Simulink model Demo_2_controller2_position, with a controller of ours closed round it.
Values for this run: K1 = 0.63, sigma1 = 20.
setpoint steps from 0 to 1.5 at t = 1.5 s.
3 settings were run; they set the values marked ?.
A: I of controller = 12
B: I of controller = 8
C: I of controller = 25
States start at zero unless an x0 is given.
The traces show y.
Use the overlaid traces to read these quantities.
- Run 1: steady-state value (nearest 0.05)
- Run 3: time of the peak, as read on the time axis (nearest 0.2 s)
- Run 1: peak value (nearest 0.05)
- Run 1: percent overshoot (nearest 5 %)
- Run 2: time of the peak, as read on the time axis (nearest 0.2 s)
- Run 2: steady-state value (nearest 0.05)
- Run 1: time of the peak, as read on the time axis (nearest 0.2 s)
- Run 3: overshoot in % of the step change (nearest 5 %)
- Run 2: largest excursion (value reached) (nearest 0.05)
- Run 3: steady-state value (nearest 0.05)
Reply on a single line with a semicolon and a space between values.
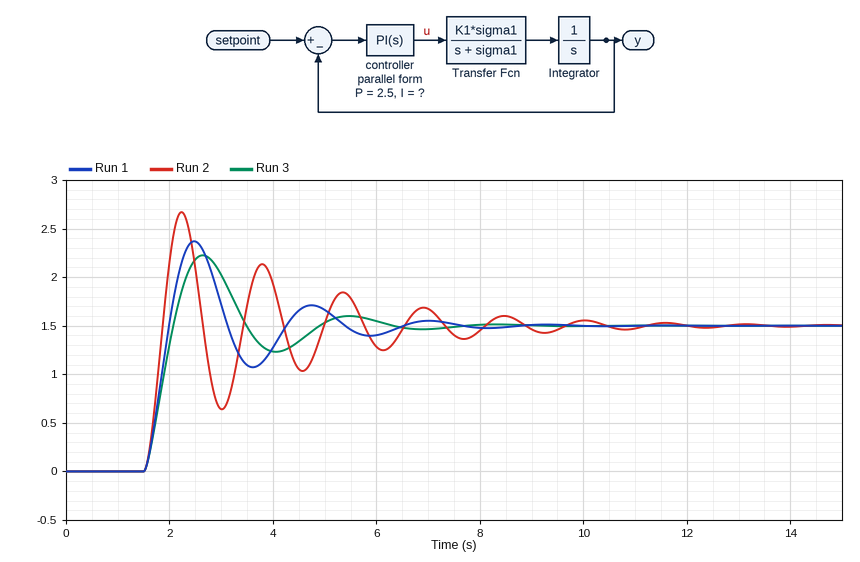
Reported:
1.50; 2.6 s; 2.35; 60 %; 2.2 s; 1.50; 2.4 s; 50 %; 2.65; 1.50
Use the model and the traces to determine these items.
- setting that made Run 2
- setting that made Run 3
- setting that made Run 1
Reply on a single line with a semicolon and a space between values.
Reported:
C; B; A
